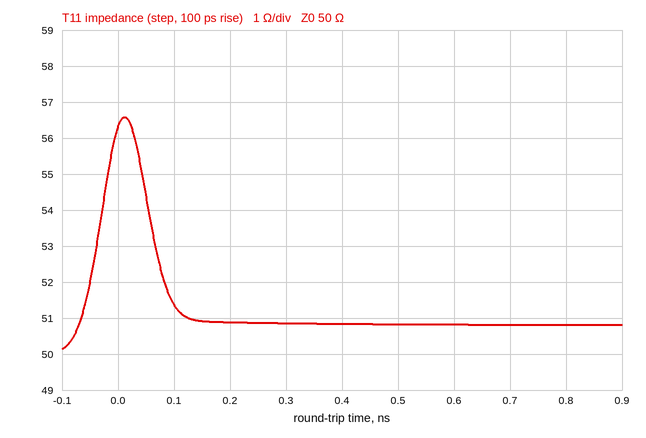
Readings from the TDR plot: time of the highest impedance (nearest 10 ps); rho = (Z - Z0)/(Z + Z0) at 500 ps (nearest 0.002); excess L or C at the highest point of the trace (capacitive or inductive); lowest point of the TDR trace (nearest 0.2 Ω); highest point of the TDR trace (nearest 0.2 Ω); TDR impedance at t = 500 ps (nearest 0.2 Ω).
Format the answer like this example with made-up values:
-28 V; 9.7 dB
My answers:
10 ps; +0.008; inductive; 50.2 Ω; 56.6 Ω; 50.8 Ω
